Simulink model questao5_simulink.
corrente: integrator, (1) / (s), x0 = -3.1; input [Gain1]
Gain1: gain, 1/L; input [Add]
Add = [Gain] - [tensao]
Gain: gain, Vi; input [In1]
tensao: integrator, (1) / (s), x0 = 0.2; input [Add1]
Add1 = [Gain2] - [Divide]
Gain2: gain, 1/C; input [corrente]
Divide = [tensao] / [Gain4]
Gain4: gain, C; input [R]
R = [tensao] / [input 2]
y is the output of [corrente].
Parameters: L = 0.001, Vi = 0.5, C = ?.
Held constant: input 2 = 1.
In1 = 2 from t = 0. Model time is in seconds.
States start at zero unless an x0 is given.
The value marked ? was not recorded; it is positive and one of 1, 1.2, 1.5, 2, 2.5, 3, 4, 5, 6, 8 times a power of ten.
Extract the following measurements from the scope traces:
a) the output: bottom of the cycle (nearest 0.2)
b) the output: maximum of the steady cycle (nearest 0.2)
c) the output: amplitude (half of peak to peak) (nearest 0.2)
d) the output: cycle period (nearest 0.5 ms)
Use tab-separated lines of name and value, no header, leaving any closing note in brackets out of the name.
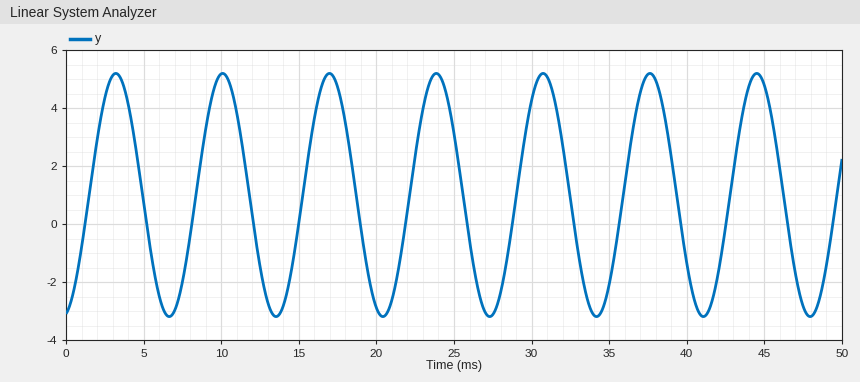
the output: bottom of the cycle	-3.2
the output: maximum of the steady cycle	5.2
the output: amplitude (half of peak to peak)	4.2
the output: cycle period	7.0 ms
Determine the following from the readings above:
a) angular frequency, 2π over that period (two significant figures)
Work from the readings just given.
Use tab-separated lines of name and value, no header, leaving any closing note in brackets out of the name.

angular frequency, 2π over that period	0.90 rad/ms
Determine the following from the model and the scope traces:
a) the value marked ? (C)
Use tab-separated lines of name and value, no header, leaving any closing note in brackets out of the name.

the value marked ?	0.0012
